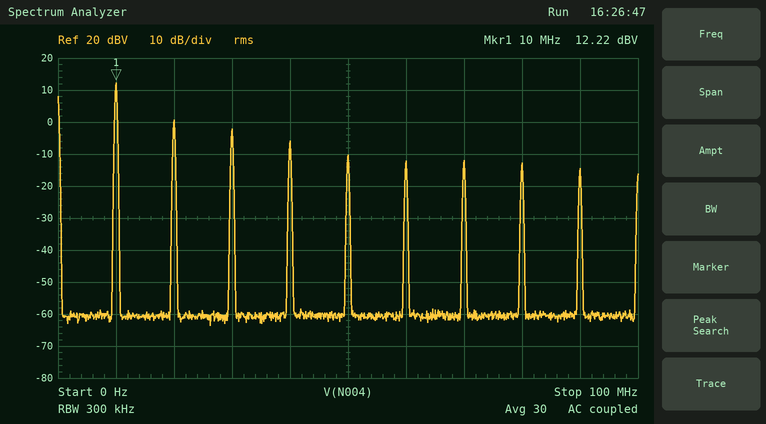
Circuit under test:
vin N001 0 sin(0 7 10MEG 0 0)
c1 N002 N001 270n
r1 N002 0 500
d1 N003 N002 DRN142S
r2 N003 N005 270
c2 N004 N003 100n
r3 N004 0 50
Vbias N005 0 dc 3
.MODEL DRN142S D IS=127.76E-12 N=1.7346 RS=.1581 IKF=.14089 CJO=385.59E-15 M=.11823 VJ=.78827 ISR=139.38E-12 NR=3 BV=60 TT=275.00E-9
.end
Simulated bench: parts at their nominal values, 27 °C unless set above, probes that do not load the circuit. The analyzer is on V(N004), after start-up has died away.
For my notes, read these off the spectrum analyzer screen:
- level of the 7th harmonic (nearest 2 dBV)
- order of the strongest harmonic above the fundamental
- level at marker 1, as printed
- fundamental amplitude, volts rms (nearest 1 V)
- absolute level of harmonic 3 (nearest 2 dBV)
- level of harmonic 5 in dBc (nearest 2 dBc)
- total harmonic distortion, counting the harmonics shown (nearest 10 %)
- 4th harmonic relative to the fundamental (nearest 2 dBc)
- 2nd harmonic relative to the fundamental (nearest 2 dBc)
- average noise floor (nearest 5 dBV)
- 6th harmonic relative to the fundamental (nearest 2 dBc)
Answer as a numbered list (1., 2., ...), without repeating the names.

1. -12 dBV
2. 2
3. 12.22 dBV
4. 4 V
5. -2 dBV
6. -22 dBc
7. 40 %
8. -18 dBc
9. -12 dBc
10. -60 dBV
11. -24 dBc
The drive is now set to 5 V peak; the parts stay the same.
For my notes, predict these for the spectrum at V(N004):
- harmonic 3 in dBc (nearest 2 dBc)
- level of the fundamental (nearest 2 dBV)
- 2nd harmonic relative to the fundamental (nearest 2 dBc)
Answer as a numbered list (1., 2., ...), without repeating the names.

1. -16 dBc
2. 10 dBV
3. -14 dBc
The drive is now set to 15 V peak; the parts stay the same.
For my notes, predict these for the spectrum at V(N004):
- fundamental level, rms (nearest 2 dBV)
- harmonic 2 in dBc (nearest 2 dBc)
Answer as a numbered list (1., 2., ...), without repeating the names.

1. 18 dBV
2. -10 dBc
